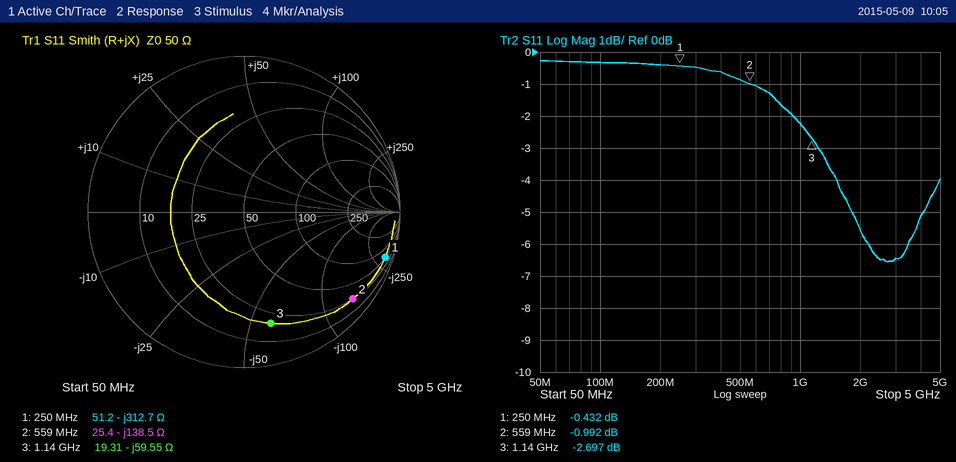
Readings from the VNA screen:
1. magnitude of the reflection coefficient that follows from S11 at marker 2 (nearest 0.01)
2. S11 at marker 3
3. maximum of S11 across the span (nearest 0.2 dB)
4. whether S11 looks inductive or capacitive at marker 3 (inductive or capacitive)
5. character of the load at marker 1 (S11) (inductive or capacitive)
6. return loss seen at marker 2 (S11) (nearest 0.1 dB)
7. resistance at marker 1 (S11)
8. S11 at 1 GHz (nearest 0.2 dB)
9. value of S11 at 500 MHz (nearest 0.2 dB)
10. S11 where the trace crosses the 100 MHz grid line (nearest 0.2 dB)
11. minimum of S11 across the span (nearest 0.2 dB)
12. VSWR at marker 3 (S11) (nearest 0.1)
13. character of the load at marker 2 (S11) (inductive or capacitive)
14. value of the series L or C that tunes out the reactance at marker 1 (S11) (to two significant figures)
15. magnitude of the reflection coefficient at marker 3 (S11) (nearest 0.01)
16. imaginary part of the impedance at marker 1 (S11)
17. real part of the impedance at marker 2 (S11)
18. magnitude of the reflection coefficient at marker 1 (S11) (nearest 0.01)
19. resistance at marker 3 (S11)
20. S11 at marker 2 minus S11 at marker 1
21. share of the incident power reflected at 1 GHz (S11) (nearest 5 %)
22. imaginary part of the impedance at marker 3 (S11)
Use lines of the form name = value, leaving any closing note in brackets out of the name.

magnitude of the reflection coefficient that follows from S11 at marker 2 = 0.89
S11 at marker 3 = -2.697 dB
maximum of S11 across the span = -0.2 dB
whether S11 looks inductive or capacitive at marker 3 = capacitive
character of the load at marker 1 (S11) = capacitive
return loss seen at marker 2 (S11) = 1.0 dB
resistance at marker 1 = 51.2 Ω
S11 at 1 GHz = -2.2 dB
value of S11 at 500 MHz = -0.8 dB
S11 where the trace crosses the 100 MHz grid line = -0.4 dB
minimum of S11 across the span = -6.6 dB
VSWR at marker 3 (S11) = 6.5
character of the load at marker 2 (S11) = capacitive
value of the series L or C that tunes out the reactance at marker 1 (S11) = 200 nH
magnitude of the reflection coefficient at marker 3 (S11) = 0.73
imaginary part of the impedance at marker 1 = -312.7 Ω
real part of the impedance at marker 2 = 25.4 Ω
magnitude of the reflection coefficient at marker 1 (S11) = 0.95
resistance at marker 3 = 19.31 Ω
S11 at marker 2 minus S11 at marker 1 = -0.560 dB
share of the incident power reflected at 1 GHz (S11) = 60 %
imaginary part of the impedance at marker 3 = -59.55 Ω
